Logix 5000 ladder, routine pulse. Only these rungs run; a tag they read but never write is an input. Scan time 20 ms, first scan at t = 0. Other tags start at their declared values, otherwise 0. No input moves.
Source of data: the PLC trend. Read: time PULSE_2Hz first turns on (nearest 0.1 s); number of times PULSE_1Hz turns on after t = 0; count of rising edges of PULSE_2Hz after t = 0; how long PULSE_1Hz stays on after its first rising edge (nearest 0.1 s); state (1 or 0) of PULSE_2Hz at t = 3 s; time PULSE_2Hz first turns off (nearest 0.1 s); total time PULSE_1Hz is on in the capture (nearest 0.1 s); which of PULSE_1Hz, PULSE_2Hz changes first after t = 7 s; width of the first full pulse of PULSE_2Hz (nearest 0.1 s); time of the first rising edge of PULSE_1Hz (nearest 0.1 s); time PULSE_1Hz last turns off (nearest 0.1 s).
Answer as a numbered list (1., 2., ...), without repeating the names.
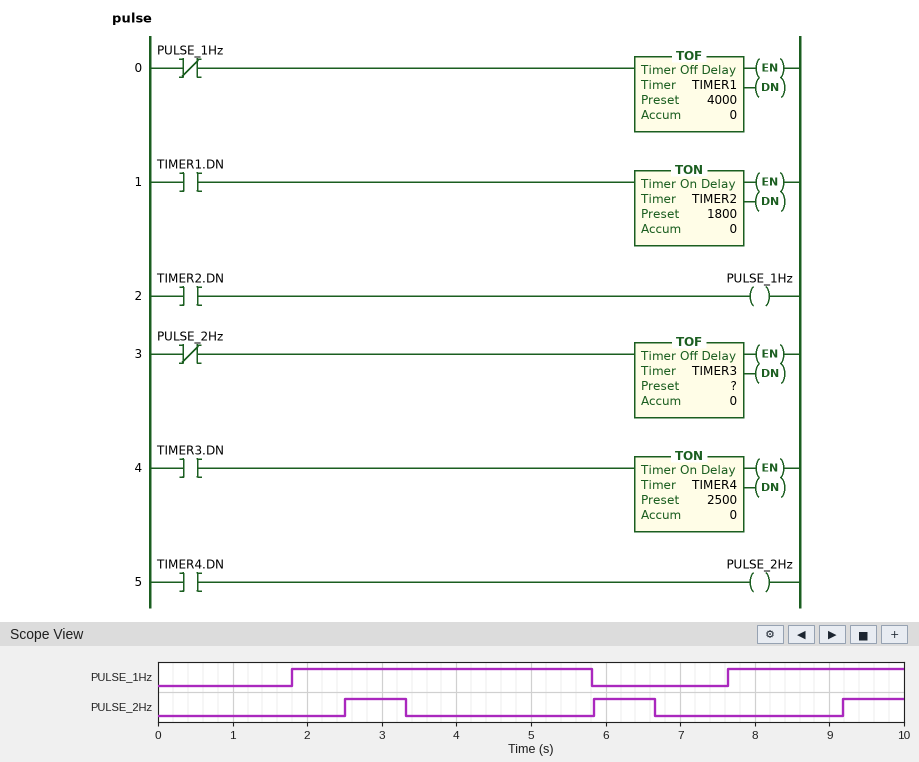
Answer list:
1. 2.5 s
2. 2
3. 3
4. 4.0 s
5. 1
6. 3.3 s
7. 6.4 s
8. PULSE_1Hz
9. 0.8 s
10. 1.8 s
11. 5.8 s
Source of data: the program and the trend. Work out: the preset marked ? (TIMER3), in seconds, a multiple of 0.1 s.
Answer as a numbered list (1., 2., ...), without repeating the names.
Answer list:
1. 0.8 s
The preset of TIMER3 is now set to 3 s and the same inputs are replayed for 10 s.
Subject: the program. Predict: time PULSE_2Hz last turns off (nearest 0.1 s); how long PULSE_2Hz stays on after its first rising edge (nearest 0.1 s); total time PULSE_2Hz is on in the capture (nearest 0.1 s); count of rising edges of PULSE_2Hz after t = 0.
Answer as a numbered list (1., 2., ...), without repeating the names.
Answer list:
1. 5.5 s
2. 3.0 s
3. 5.0 s
4. 2
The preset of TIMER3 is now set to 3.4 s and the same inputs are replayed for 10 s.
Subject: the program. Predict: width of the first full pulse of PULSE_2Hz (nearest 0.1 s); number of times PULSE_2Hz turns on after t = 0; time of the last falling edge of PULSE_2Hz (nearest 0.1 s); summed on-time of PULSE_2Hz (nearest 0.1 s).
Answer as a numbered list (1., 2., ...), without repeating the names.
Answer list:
1. 3.4 s
2. 2
3. 5.9 s
4. 5.0 s
